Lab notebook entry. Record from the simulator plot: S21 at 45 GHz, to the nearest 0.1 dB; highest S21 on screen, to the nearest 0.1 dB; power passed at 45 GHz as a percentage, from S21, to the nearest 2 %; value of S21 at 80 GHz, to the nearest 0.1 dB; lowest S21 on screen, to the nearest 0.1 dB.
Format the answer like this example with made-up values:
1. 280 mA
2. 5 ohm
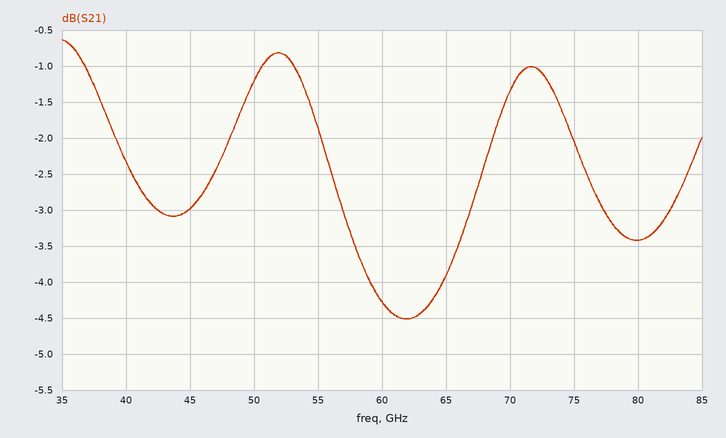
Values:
1. -3.0 dB
2. -0.6 dB
3. 50 %
4. -3.4 dB
5. -4.5 dB
